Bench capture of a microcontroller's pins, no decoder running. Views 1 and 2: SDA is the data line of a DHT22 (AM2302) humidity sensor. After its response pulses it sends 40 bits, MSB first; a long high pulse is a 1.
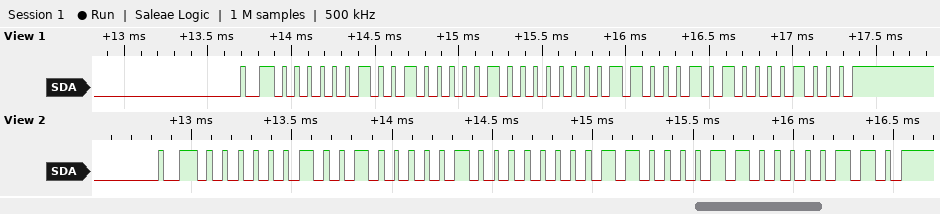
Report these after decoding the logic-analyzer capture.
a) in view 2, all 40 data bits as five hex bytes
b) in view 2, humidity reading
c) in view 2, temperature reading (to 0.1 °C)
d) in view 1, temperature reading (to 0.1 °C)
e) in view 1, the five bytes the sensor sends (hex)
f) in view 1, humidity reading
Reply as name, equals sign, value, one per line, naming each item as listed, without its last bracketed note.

in view 2, all 40 data bits as five hex bytes = 02 41 00 C3 06
in view 2, humidity reading = 57.7 %
in view 2, temperature reading = 19.5 °C
in view 1, temperature reading = 19.7 °C
in view 1, the five bytes the sensor sends = 02 41 00 C5 08
in view 1, humidity reading = 57.7 %
